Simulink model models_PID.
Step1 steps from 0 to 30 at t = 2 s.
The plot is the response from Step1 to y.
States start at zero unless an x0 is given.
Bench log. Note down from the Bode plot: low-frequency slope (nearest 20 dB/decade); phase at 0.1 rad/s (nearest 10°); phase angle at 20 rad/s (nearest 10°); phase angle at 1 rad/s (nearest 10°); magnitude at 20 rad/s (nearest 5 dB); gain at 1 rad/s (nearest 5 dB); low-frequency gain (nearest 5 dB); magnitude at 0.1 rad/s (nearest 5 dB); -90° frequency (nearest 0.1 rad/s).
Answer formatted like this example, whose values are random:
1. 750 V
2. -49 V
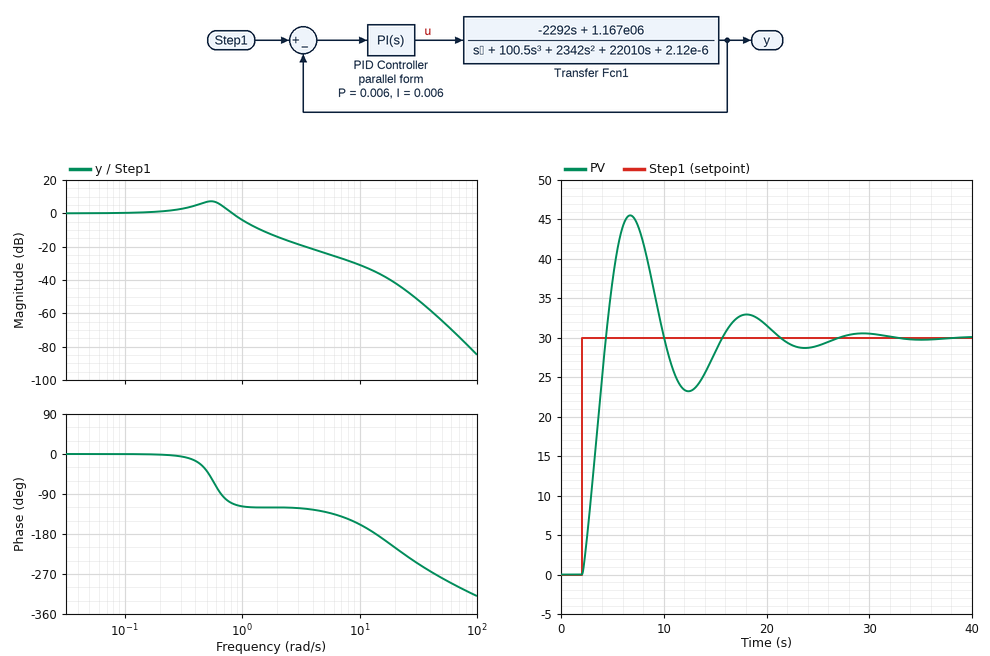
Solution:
1. 0 dB/decade
2. 0°
3. -210°
4. -120°
5. -40 dB
6. -5 dB
7. 0 dB
8. 0 dB
9. 0.7 rad/s
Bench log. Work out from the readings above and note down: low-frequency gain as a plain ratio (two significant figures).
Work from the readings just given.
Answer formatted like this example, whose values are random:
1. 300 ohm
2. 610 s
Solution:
1. 1.0
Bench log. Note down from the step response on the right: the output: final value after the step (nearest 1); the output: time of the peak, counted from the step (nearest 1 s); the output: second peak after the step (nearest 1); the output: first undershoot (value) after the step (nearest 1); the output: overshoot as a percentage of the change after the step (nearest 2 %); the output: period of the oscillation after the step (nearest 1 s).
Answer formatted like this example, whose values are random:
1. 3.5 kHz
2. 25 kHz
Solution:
1. 30
2. 5 s
3. 33
4. 23
5. 52 %
6. 11 s
